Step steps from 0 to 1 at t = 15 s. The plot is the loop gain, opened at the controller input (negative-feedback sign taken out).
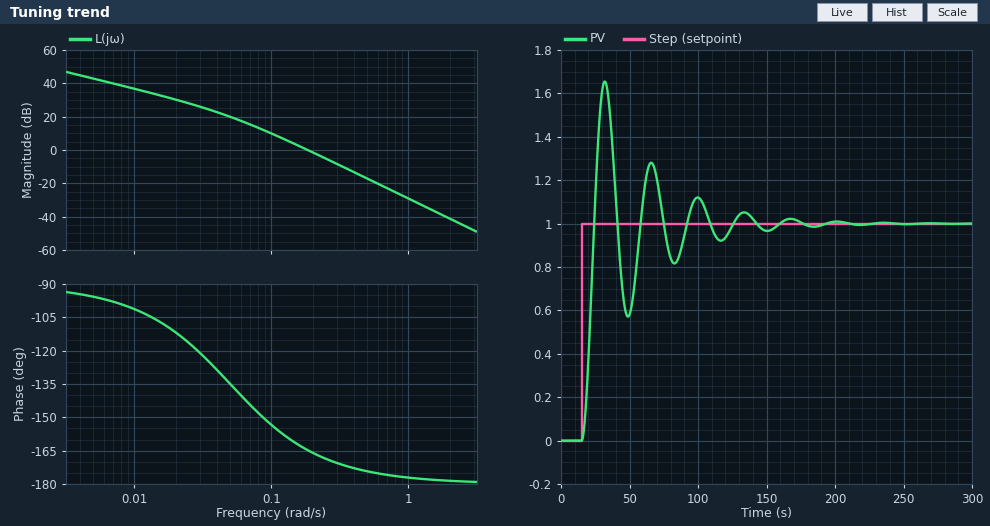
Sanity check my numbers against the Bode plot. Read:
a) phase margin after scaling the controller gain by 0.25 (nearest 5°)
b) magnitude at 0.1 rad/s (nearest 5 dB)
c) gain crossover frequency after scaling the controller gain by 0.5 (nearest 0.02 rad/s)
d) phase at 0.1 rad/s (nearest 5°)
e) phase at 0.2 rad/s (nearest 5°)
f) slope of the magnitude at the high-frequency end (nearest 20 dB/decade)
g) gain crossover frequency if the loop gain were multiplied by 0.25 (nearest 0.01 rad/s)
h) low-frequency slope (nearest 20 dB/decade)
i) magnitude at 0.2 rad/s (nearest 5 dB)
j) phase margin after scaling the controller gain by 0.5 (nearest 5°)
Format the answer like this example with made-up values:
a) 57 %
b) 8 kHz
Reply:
a) 30°
b) 10 dB
c) 0.12 rad/s
d) -155°
e) -165°
f) -40 dB/decade
g) 0.09 rad/s
h) -20 dB/decade
i) 0 dB
j) 20°
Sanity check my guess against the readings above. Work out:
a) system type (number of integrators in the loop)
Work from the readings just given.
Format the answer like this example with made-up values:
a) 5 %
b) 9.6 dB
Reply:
a) 1
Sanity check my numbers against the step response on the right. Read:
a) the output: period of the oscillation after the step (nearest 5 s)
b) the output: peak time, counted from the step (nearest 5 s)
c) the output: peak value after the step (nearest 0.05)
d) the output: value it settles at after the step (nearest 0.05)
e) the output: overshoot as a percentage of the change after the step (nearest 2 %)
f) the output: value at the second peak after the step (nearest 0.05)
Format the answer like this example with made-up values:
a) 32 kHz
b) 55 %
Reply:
a) 35 s
b) 15 s
c) 1.65
d) 1.00
e) 66 %
f) 1.30
